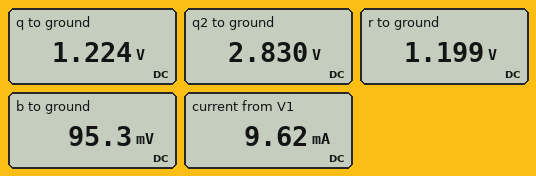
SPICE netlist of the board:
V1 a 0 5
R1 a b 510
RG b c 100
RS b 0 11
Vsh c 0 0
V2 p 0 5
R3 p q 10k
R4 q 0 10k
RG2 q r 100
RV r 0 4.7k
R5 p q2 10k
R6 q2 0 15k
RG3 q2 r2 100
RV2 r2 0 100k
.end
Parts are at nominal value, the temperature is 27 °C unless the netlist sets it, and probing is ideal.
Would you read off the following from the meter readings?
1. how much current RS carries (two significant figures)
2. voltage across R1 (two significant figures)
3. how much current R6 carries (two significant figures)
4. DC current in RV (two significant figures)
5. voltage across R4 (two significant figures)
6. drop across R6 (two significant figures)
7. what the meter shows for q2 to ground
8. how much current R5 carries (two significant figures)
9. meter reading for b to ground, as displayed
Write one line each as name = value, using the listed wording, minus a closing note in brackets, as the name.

how much current RS carries = 8.7 mA
voltage across R1 = 4.9 V
how much current R6 carries = 190 µA
DC current in RV = 260 µA
voltage across R4 = 1.2 V
drop across R6 = 2.8 V
what the meter shows for q2 to ground = 2.830 V
how much current R5 carries = 220 µA
meter reading for b to ground, as displayed = 95.3 mV
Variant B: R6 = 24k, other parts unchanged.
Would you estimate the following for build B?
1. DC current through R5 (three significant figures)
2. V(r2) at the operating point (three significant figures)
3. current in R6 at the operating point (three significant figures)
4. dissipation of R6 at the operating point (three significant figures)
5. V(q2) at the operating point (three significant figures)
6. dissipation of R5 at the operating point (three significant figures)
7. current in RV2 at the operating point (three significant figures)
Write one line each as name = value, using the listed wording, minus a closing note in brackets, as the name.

DC current through R5 = 170 µA
V(r2) at the operating point = 3.29 V
current in R6 at the operating point = 137 µA
dissipation of R6 at the operating point = 453 µW
V(q2) at the operating point = 3.30 V
dissipation of R5 at the operating point = 290 µW
current in RV2 at the operating point = 32.9 µA
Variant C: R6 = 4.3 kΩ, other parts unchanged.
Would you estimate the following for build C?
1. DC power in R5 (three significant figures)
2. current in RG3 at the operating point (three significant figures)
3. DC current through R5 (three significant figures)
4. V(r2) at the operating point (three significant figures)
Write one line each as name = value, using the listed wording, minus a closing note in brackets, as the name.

DC power in R5 = 1.25 mW
current in RG3 at the operating point = 14.6 µA
DC current through R5 = 354 µA
V(r2) at the operating point = 1.46 V
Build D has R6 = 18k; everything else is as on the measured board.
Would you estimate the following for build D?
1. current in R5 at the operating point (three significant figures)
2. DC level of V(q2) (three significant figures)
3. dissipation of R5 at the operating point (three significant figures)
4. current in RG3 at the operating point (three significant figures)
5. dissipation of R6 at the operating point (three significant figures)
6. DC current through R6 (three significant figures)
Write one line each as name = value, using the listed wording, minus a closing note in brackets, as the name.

current in R5 at the operating point = 198 µA
DC level of V(q2) = 3.02 V
dissipation of R5 at the operating point = 392 µW
current in RG3 at the operating point = 30.2 µA
dissipation of R6 at the operating point = 507 µW
DC current through R6 = 168 µA
